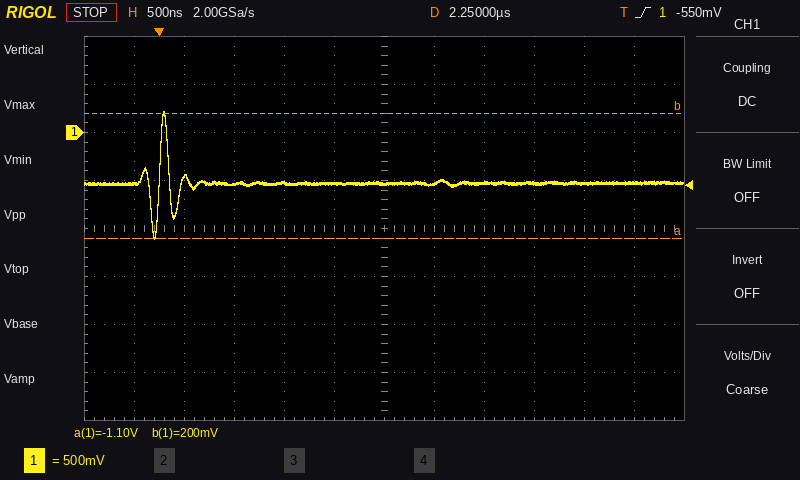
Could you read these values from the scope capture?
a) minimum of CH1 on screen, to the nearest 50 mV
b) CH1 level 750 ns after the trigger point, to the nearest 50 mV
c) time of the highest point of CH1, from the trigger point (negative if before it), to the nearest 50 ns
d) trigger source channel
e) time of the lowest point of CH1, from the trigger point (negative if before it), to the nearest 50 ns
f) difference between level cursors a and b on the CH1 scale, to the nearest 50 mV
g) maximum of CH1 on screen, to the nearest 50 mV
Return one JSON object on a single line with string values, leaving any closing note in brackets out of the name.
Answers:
{"minimum of CH1 on screen, to the nearest 50 mV": "-1.10 V", "CH1 level 750 ns after the trigger point, to the nearest 50 mV": "-550 mV", "time of the highest point of CH1, from the trigger point (negative if before it), to the nearest 50 ns": "+50 ns", "trigger source channel": "CH1", "time of the lowest point of CH1, from the trigger point (negative if before it), to the nearest 50 ns": "-50 ns", "difference between level cursors a and b on the CH1 scale, to the nearest 50 mV": "1.30 V", "maximum of CH1 on screen, to the nearest 50 mV": "200 mV"}
